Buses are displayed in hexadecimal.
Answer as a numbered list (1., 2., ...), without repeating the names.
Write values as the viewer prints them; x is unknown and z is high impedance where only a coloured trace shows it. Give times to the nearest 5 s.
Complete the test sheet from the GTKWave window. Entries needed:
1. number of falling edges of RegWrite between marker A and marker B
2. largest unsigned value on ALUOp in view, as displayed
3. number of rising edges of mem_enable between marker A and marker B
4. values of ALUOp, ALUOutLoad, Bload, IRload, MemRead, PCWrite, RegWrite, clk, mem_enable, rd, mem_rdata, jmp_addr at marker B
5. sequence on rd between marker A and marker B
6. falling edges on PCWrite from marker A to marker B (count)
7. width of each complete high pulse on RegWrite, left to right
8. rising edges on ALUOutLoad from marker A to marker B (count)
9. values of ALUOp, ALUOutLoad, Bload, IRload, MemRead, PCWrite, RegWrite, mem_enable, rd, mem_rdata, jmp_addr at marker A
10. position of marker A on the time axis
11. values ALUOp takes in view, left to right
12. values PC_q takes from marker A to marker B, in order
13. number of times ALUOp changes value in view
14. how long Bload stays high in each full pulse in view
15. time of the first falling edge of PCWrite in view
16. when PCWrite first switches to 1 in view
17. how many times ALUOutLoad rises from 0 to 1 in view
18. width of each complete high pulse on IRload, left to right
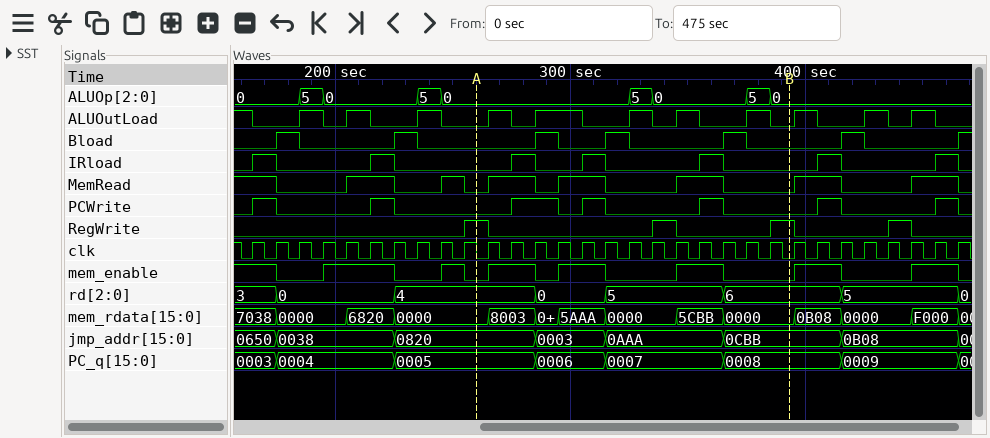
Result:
1. 2
2. 5
3. 3
4. ALUOp=0, ALUOutLoad=0, Bload=0, IRload=0, MemRead=0, PCWrite=0, RegWrite=1, clk=0, mem_enable=0, rd=6, mem_rdata=0000, jmp_addr=0CBB
5. 4, 0, 5, 6
6. 3
7. 10 s, 10 s, 10 s, 10 s
8. 5
9. ALUOp=0, ALUOutLoad=0, Bload=0, IRload=0, MemRead=0, PCWrite=0, RegWrite=1, mem_enable=0, rd=4, mem_rdata=0000, jmp_addr=0820
10. 260 s
11. 0, 5, 0, 5, 0, 5, 0, 5, 0
12. 0005, 0006, 0007, 0008
13. 8
14. 10 s, 10 s, 10 s, 10 s, 10 s, 10 s
15. 175 s
16. 165 s
17. 11
18. 10 s, 10 s, 10 s, 10 s, 10 s, 10 s, 10 s
